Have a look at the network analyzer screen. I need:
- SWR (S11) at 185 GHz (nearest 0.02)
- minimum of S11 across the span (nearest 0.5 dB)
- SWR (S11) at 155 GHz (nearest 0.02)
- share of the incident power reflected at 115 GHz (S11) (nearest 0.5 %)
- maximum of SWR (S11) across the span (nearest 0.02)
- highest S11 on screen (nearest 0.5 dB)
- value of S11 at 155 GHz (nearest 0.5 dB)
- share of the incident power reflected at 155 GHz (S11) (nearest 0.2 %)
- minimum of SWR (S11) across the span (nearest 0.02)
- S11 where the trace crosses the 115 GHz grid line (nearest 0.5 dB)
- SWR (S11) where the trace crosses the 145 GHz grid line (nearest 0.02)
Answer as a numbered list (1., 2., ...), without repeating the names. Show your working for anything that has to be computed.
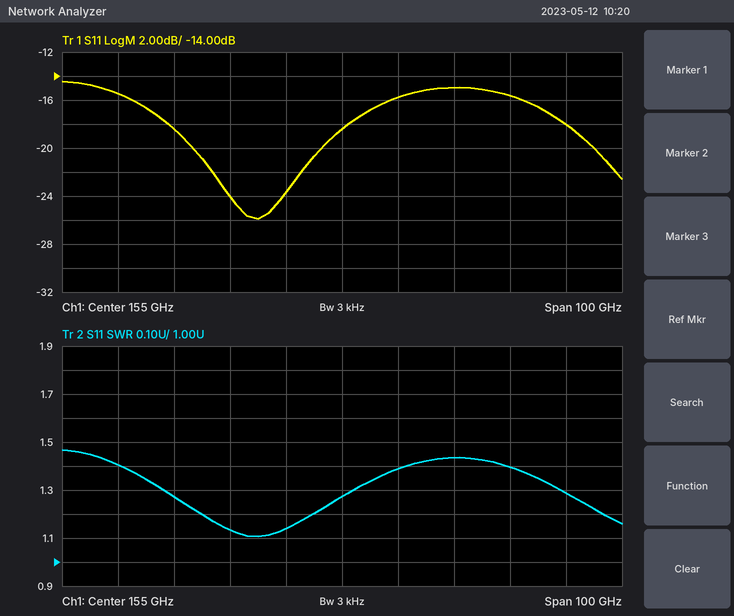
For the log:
1. 1.40
2. -26.0 dB
3. 1.28
4. 10^(-15.5/10) ≈ 2.82 %, so 3.0 % to the nearest 0.5 %
5. 1.46
6. -14.5 dB
7. -18.5 dB
8. 10^(-18.5/10) ≈ 1.4 %
9. 1.10
10. -15.5 dB
11. 1.14
